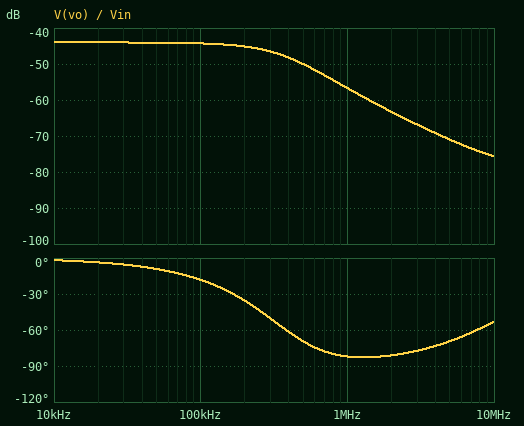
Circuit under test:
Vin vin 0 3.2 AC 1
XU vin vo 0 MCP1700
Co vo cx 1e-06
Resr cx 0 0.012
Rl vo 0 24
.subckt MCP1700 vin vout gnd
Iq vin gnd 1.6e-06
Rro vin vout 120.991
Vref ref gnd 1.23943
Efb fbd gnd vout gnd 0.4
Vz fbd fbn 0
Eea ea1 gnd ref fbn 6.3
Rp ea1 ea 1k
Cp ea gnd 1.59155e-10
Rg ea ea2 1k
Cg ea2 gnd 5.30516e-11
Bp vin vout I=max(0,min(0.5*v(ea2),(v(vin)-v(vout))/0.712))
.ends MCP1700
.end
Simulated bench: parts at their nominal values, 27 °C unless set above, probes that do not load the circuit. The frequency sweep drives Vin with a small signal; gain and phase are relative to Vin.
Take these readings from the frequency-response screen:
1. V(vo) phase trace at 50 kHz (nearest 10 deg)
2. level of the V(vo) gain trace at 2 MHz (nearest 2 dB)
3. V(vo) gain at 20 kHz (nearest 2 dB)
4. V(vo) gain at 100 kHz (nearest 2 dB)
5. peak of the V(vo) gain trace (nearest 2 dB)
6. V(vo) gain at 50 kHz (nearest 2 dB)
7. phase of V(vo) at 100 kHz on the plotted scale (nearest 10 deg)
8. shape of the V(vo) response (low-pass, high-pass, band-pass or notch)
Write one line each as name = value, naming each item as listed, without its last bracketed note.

V(vo) phase trace at 50 kHz = -10 deg
level of the V(vo) gain trace at 2 MHz = -64 dB
V(vo) gain at 20 kHz = -44 dB
V(vo) gain at 100 kHz = -44 dB
peak of the V(vo) gain trace = -44 dB
V(vo) gain at 50 kHz = -44 dB
phase of V(vo) at 100 kHz on the plotted scale = -20 deg
shape of the V(vo) response = low-pass
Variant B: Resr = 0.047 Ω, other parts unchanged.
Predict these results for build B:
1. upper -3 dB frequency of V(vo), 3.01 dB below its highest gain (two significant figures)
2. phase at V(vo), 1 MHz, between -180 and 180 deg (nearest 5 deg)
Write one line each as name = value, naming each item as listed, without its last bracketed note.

upper -3 dB frequency of V(vo), 3.01 dB below its highest gain = 310 kHz
phase at V(vo), 1 MHz, between -180 and 180 deg = -70 deg
